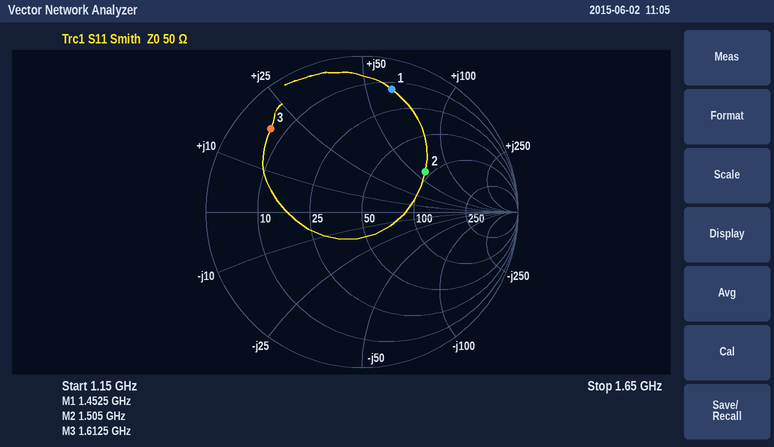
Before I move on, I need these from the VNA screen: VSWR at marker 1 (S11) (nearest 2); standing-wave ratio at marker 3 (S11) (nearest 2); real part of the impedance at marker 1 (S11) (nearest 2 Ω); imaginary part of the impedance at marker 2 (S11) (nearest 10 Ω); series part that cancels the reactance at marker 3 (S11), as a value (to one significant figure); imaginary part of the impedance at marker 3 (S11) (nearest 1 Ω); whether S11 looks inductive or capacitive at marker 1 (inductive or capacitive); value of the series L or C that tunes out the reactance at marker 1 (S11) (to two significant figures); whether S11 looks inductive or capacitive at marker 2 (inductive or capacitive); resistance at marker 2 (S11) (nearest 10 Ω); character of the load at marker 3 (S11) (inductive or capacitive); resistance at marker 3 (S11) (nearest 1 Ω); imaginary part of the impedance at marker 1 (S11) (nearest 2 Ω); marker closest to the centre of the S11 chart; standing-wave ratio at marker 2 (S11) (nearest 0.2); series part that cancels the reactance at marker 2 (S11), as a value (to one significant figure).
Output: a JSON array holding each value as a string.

["10", "8", "14 Ω", "+60 Ω", "5 pF", "+19 Ω", "inductive", "1.8 pF", "inductive", "90 Ω", "inductive", "7 Ω", "+62 Ω", "marker 2", "2.8", "2 pF"]
